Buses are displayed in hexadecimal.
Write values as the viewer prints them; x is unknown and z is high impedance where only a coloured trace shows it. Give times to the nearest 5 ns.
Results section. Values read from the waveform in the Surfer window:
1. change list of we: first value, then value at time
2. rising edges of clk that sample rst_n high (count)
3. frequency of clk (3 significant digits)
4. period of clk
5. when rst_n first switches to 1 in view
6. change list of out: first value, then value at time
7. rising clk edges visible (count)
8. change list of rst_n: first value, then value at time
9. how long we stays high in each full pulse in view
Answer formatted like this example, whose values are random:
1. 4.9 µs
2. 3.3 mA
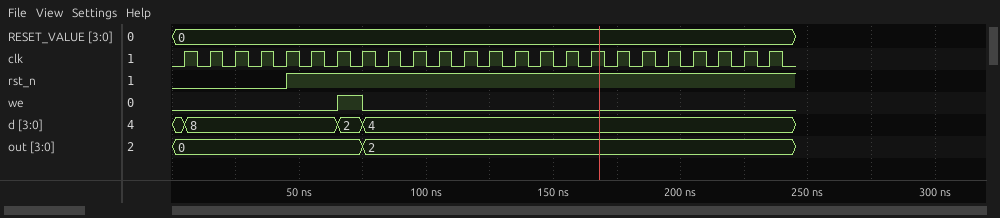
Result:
1. 0, 1 at 65 ns, 0 at 75 ns
2. 19
3. 100 MHz
4. 10 ns
5. 45 ns
6. 0, 2 at 75 ns
7. 24
8. 0, 1 at 45 ns
9. 10 ns
